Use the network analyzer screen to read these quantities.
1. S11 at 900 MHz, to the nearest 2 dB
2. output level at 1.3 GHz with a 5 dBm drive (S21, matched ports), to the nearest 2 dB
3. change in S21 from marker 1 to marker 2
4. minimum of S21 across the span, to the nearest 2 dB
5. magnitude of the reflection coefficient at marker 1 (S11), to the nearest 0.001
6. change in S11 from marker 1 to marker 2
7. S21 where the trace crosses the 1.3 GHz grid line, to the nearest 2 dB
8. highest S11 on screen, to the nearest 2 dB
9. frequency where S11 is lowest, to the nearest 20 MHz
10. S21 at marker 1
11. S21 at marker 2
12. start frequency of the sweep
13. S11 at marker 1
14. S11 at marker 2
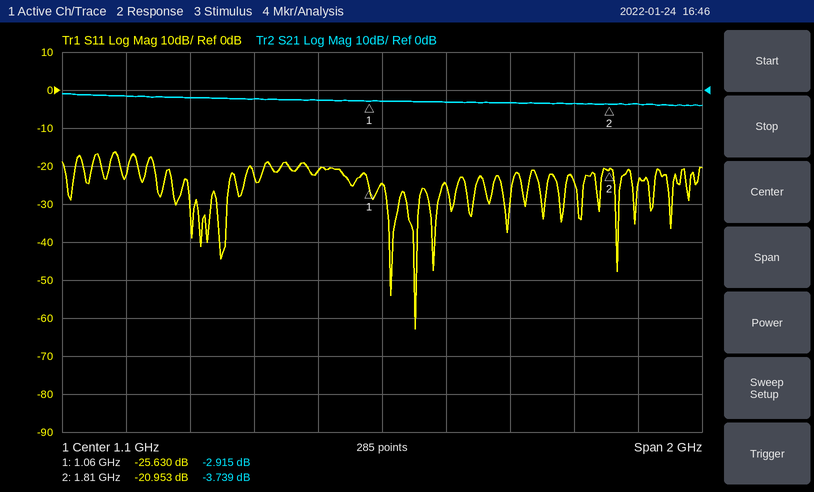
-22 dB
2 dBm
-0.824 dB
-4 dB
0.052
4.677 dB
-4 dB
-16 dB
1.20 GHz
-2.915 dB
-3.739 dB
100 MHz
-25.630 dB
-20.953 dB
